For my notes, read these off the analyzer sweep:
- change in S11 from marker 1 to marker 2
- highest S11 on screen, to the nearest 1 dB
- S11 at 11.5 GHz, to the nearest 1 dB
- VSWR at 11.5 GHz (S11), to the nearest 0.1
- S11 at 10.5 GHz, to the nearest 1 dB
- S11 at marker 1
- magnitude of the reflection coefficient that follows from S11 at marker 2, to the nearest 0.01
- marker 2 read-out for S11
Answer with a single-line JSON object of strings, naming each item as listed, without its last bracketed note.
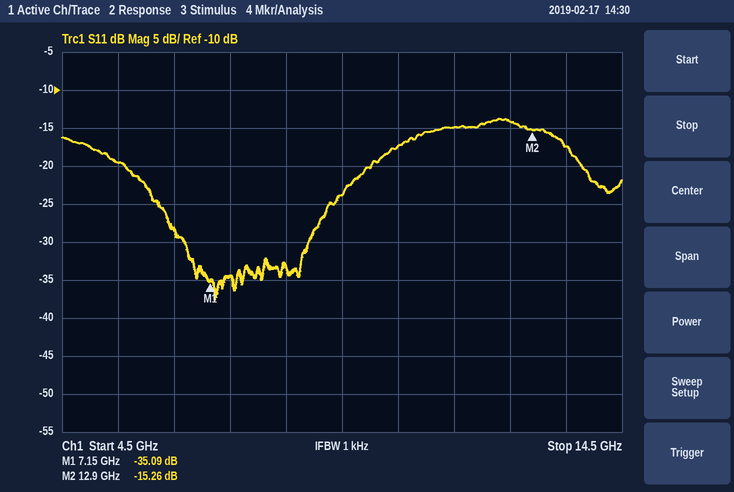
{"change in S11 from marker 1 to marker 2": "19.83 dB", "highest S11 on screen, to the nearest 1 dB": "-14 dB", "S11 at 11.5 GHz, to the nearest 1 dB": "-15 dB", "VSWR at 11.5 GHz (S11), to the nearest 0.1": "1.4", "S11 at 10.5 GHz, to the nearest 1 dB": "-17 dB", "S11 at marker 1": "-35.09 dB", "magnitude of the reflection coefficient that follows from S11 at marker 2, to the nearest 0.01": "0.17", "marker 2 read-out for S11": "-15.26 dB"}
